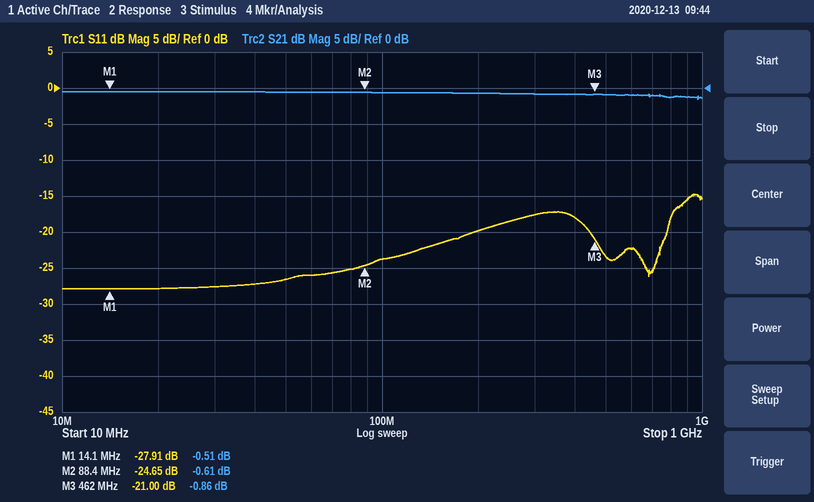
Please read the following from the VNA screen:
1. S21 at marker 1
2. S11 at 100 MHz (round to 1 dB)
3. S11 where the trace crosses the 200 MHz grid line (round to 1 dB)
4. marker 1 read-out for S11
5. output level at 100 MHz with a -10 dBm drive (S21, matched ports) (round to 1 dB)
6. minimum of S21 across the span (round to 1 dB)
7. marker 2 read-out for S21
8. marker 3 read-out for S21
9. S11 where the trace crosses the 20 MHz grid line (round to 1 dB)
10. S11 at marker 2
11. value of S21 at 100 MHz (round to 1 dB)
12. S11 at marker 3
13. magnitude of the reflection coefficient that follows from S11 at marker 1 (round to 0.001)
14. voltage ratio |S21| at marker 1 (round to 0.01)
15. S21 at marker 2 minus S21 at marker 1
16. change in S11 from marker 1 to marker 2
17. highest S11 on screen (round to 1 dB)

-0.51 dB
-24 dB
-20 dB
-27.91 dB
-11 dBm
-2 dB
-0.61 dB
-0.86 dB
-28 dB
-24.65 dB
-1 dB
-21.00 dB
0.040
0.94
-0.10 dB
3.26 dB
-15 dB
